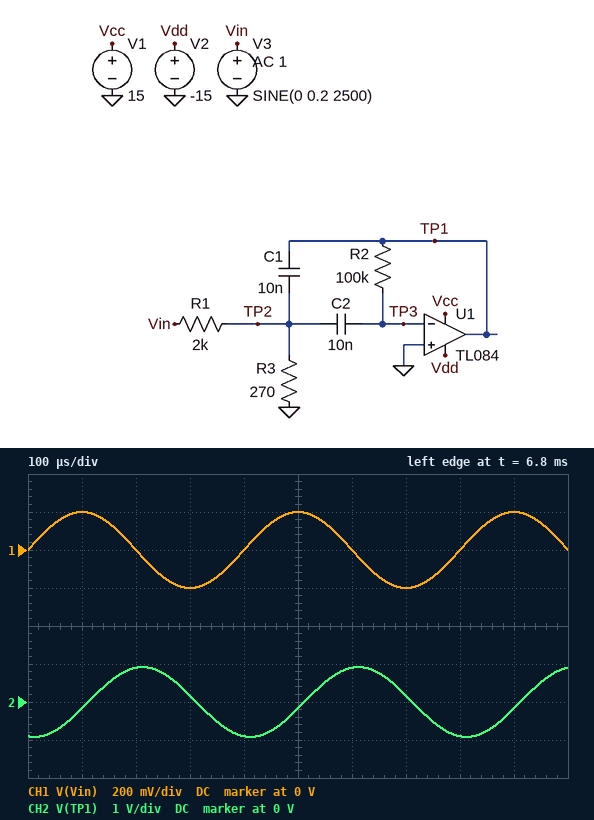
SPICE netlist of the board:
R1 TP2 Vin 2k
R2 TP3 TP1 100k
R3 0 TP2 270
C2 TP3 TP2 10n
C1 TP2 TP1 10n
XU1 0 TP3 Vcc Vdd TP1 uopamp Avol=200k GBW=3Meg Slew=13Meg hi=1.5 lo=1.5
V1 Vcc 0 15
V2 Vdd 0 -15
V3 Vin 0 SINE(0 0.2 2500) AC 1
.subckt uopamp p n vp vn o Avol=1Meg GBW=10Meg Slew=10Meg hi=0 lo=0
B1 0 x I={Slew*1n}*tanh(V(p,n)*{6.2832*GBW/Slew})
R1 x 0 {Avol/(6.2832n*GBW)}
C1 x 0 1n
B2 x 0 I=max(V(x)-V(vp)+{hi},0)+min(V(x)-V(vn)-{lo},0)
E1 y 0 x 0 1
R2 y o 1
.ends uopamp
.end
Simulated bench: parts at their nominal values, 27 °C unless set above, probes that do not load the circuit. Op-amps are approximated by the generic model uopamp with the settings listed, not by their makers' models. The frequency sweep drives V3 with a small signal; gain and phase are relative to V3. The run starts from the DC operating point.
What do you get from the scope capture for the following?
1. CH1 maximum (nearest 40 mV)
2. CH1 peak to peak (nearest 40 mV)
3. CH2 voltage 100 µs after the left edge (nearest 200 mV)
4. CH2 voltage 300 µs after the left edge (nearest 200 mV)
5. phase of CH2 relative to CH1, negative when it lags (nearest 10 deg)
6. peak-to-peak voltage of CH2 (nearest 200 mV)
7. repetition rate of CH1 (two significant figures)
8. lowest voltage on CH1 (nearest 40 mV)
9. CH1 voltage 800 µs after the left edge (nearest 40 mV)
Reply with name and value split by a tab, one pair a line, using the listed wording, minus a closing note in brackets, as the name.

CH1 maximum	200 mV
CH1 peak to peak	400 mV
CH2 voltage 100 µs after the left edge	-200 mV
CH2 voltage 300 µs after the left edge	200 mV
phase of CH2 relative to CH1, negative when it lags	-100 deg
peak-to-peak voltage of CH2	1.8 V
repetition rate of CH1	2.5 kHz
lowest voltage on CH1	-200 mV
CH1 voltage 800 µs after the left edge	0 V
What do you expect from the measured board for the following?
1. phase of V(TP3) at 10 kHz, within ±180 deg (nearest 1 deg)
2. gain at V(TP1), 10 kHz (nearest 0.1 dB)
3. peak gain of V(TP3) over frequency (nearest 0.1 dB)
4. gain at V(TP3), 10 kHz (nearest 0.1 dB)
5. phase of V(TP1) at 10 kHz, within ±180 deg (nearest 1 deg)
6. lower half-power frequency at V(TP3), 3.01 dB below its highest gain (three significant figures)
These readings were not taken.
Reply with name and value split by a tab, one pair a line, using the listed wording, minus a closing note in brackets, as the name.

phase of V(TP3) at 10 kHz, within ±180 deg	2 deg
gain at V(TP1), 10 kHz	-1.2 dB
peak gain of V(TP3) over frequency	-31.4 dB
gain at V(TP3), 10 kHz	-50.8 dB
phase of V(TP1) at 10 kHz, within ±180 deg	92 deg
lower half-power frequency at V(TP3), 3.01 dB below its highest gain	3.09 kHz
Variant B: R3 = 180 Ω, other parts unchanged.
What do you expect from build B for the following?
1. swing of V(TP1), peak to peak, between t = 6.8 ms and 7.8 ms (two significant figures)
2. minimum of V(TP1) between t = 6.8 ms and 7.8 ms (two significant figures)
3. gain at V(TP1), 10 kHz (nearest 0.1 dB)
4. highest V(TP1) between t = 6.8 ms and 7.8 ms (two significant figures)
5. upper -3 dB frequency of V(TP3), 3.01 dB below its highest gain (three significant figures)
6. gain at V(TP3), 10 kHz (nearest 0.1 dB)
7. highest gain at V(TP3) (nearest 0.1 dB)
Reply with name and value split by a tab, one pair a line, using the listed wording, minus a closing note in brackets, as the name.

swing of V(TP1), peak to peak, between t = 6.8 ms and 7.8 ms	890 mV
minimum of V(TP1) between t = 6.8 ms and 7.8 ms	-450 mV
gain at V(TP1), 10 kHz	-0.9 dB
highest V(TP1) between t = 6.8 ms and 7.8 ms	450 mV
upper -3 dB frequency of V(TP3), 3.01 dB below its highest gain	4.03 kHz
gain at V(TP3), 10 kHz	-50.4 dB
highest gain at V(TP3)	-29.9 dB
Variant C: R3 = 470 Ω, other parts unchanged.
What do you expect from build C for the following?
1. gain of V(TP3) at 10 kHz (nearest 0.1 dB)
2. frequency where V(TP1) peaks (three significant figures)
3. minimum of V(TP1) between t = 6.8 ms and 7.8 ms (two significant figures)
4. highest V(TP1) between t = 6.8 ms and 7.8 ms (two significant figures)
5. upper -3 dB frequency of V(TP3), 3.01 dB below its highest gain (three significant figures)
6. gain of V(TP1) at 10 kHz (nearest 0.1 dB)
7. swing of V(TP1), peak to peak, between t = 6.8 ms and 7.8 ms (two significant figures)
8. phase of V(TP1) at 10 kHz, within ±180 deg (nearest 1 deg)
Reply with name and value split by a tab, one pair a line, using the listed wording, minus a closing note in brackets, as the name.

gain of V(TP3) at 10 kHz	-51.1 dB
frequency where V(TP1) peaks	2.56 kHz
minimum of V(TP1) between t = 6.8 ms and 7.8 ms	-4.6 V
highest V(TP1) between t = 6.8 ms and 7.8 ms	4.6 V
upper -3 dB frequency of V(TP3), 3.01 dB below its highest gain	2.75 kHz
gain of V(TP1) at 10 kHz	-1.5 dB
swing of V(TP1), peak to peak, between t = 6.8 ms and 7.8 ms	9.3 V
phase of V(TP1) at 10 kHz, within ±180 deg	92 deg
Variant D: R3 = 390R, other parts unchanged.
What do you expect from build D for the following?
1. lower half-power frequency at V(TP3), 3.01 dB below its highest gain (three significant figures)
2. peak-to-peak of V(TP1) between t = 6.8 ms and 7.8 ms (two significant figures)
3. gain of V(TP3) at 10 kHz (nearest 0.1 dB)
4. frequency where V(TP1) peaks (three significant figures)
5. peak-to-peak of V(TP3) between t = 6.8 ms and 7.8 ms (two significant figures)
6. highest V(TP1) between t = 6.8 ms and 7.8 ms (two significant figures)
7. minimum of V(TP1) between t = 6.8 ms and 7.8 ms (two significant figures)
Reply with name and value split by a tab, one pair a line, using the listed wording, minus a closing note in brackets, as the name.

lower half-power frequency at V(TP3), 3.01 dB below its highest gain	2.63 kHz
peak-to-peak of V(TP1) between t = 6.8 ms and 7.8 ms	4.9 V
gain of V(TP3) at 10 kHz	-51.0 dB
frequency where V(TP1) peaks	2.76 kHz
peak-to-peak of V(TP3) between t = 6.8 ms and 7.8 ms	4.1 mV
highest V(TP1) between t = 6.8 ms and 7.8 ms	2.5 V
minimum of V(TP1) between t = 6.8 ms and 7.8 ms	-2.5 V
